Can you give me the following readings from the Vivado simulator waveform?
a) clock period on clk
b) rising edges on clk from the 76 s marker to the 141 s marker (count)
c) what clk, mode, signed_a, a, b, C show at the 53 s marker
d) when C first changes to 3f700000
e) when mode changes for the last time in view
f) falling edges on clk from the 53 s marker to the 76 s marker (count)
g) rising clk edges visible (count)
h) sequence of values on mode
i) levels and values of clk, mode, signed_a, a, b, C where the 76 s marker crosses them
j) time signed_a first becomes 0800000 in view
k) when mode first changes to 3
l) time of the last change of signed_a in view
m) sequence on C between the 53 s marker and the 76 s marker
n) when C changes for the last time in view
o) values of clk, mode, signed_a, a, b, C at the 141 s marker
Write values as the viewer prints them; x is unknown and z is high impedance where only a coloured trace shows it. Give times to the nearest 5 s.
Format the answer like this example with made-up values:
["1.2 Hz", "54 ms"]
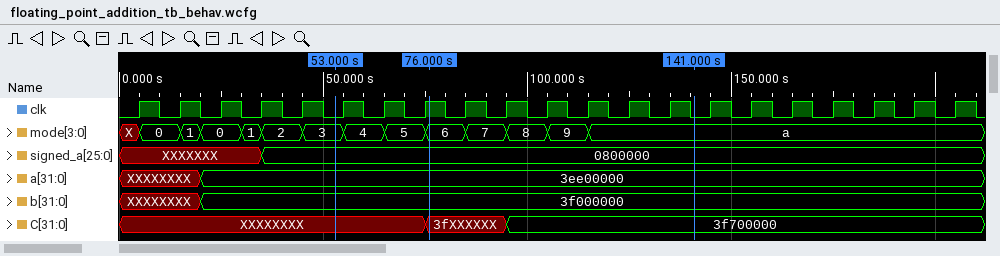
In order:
["10 s", "6", "clk=0, mode=3, signed_a=0800000, a=3ee00000, b=3f000000, C=XXXXXXXX", "95 s", "115 s", "2", "21", "X, 0, 1, 0, 1, 2, 3, 4, 5, 6, 7, 8, 9, a", "clk=1, mode=6, signed_a=0800000, a=3ee00000, b=3f000000, C=3fXXXXXX", "35 s", "45 s", "35 s", "XXXXXXXX, 3fXXXXXX", "95 s", "clk=0, mode=a, signed_a=0800000, a=3ee00000, b=3f000000, C=3f700000"]
